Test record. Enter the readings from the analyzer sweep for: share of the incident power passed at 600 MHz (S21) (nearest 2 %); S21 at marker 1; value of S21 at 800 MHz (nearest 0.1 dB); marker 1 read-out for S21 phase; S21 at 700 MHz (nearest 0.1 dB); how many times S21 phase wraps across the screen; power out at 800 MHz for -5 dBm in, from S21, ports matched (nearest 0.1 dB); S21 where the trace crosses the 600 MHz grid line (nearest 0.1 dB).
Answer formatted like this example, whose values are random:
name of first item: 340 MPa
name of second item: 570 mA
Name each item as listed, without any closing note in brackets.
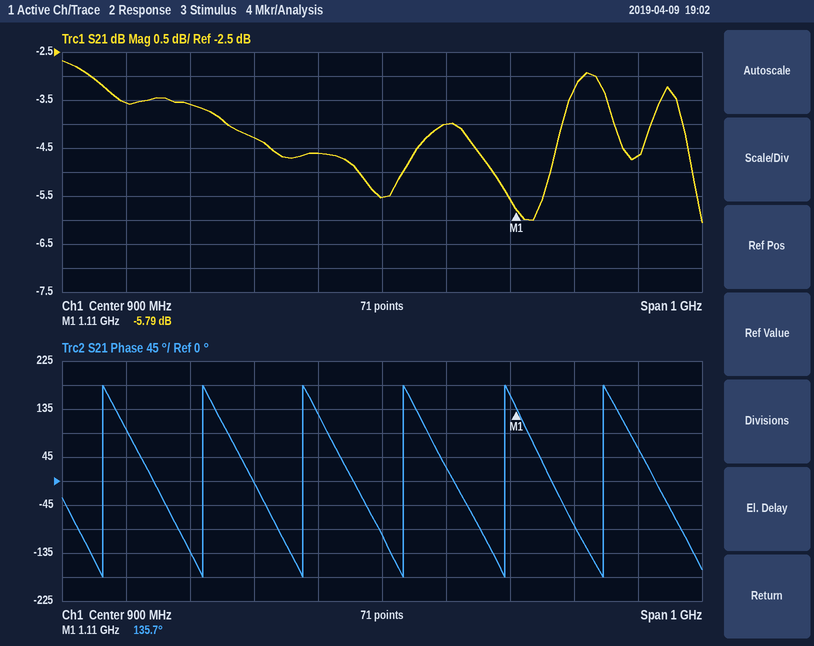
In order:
share of the incident power passed at 600 MHz (S21): 44 %
S21 at marker 1: -5.79 dB
value of S21 at 800 MHz: -4.6 dB
marker 1 read-out for S21 phase: 135.7°
S21 at 700 MHz: -4.3 dB
how many times S21 phase wraps across the screen: 6
power out at 800 MHz for -5 dBm in, from S21, ports matched: -9.6 dBm
S21 where the trace crosses the 600 MHz grid line: -3.6 dB
